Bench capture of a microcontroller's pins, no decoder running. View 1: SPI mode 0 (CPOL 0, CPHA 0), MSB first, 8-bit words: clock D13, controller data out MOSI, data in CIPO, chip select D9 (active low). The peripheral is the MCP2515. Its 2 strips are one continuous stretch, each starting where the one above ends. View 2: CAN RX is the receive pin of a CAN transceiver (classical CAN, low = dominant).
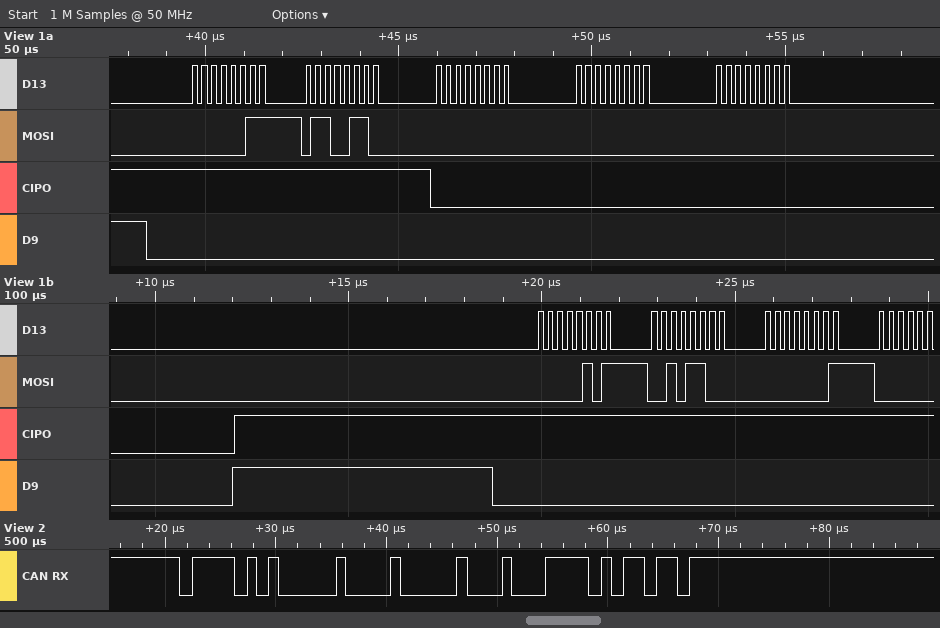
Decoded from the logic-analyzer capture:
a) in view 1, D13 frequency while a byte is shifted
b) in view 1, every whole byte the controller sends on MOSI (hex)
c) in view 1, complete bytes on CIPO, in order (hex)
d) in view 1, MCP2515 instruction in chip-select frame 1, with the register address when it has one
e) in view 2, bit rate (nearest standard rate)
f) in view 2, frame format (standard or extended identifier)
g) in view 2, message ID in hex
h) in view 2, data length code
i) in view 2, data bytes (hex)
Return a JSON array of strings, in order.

["4 MHz", "03 66 00 00 00 05 2C 01", "FF FF 00 00 00 FF FF FF", "READ 0x66", "1000 kbit/s", "standard", "0x7A8", "1", "00"]
